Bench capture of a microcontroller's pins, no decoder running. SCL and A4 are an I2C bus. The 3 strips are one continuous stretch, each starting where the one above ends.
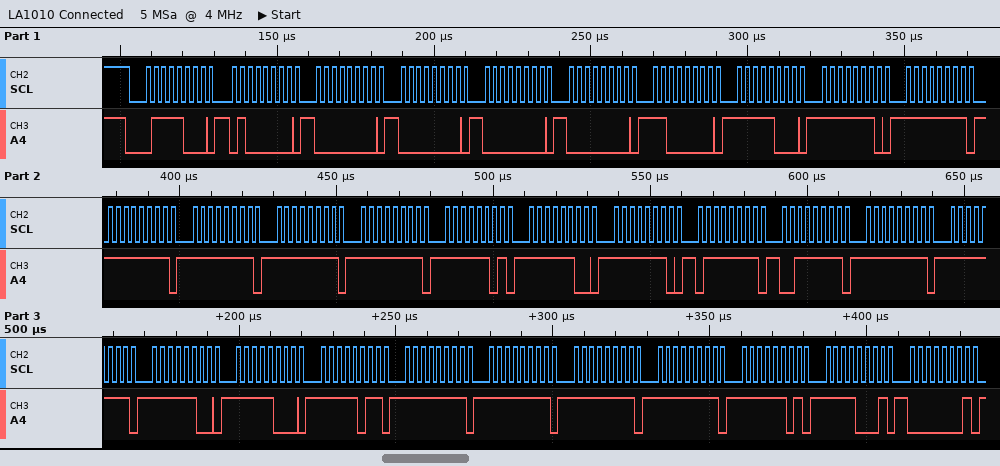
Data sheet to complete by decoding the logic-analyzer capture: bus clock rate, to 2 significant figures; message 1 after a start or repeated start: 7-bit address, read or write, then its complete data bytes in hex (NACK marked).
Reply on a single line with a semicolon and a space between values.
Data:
400 kHz; 0x3C write: 40 00 00 00 00 C0 F8 FE FF FF FF FF FF FD FC FE 7F 3F FF FF FC F8 FB FF FF FF FF FD F1 01
